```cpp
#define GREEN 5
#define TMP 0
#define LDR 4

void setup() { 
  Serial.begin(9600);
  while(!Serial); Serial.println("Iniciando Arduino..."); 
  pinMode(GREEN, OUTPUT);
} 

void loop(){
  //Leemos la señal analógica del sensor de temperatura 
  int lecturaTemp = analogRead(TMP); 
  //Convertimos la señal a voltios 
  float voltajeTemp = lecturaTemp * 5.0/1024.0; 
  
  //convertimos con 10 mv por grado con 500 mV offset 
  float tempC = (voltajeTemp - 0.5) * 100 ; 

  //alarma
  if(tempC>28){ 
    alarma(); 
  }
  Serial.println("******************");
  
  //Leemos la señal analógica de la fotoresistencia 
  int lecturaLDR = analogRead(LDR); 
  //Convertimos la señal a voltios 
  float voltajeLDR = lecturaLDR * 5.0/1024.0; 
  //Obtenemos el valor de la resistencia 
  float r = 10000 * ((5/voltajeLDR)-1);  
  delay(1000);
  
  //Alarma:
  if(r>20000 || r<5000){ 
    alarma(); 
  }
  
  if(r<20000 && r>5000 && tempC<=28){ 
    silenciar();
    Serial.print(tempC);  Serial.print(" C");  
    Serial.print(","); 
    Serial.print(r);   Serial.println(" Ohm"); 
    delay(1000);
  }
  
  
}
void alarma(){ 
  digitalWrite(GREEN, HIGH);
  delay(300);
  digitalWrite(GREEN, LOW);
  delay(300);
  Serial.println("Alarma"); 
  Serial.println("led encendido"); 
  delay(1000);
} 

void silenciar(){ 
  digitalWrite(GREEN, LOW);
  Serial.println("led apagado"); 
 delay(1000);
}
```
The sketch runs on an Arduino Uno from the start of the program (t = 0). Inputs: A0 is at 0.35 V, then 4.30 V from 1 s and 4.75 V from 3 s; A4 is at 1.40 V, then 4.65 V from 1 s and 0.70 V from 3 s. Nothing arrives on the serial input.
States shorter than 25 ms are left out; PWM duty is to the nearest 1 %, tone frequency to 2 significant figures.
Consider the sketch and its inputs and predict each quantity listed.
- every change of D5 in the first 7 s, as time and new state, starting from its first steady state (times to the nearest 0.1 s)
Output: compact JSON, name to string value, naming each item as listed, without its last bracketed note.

{"every change of D5 in the first 7 s, as time and new state, starting from its first steady state": "0 s low; 1 s high; 1.3 s low; 2.6 s high; 2.9 s low; 5.2 s high; 5.5 s low; 6.8 s high"}
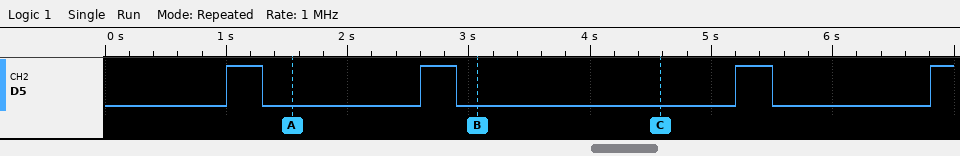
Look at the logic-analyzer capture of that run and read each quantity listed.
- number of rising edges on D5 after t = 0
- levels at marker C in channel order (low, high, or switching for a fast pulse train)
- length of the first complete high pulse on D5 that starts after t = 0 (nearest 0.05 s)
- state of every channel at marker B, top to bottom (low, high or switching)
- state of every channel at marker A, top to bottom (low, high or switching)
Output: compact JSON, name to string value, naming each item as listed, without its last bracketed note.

{"number of rising edges on D5 after t = 0": "4", "levels at marker C in channel order": "D5 low", "length of the first complete high pulse on D5 that starts after t = 0": "0.30 s", "state of every channel at marker B, top to bottom": "D5 low", "state of every channel at marker A, top to bottom": "D5 low"}
